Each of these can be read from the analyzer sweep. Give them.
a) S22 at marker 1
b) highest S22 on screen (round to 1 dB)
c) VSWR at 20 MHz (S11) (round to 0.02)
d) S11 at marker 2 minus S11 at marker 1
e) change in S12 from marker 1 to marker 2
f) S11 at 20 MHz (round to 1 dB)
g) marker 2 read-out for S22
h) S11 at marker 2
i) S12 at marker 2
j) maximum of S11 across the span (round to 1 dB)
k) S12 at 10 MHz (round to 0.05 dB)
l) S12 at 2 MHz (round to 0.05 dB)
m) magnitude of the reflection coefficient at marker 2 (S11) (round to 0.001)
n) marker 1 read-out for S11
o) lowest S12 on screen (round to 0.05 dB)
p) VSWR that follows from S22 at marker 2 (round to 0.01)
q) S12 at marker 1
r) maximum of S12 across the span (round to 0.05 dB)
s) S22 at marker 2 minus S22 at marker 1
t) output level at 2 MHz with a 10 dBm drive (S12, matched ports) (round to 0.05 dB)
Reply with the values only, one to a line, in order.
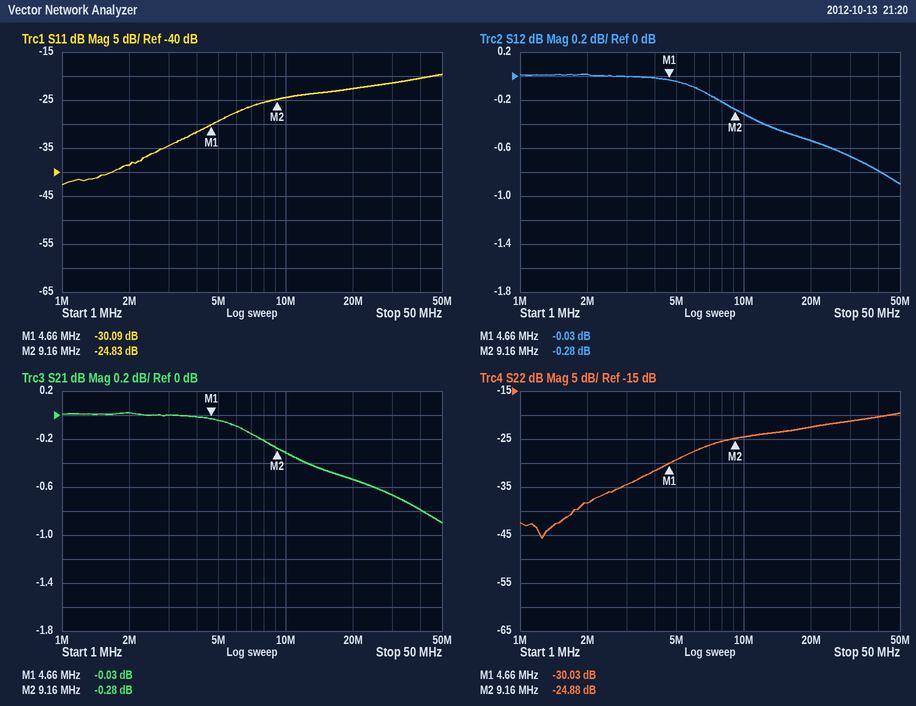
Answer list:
-30.03 dB
-20 dB
1.16
5.26 dB
-0.25 dB
-23 dB
-24.88 dB
-24.83 dB
-0.28 dB
-20 dB
-0.30 dB
0.00 dB
0.057
-30.09 dB
-0.90 dB
1.12
-0.03 dB
0.00 dB
5.15 dB
10.00 dBm
